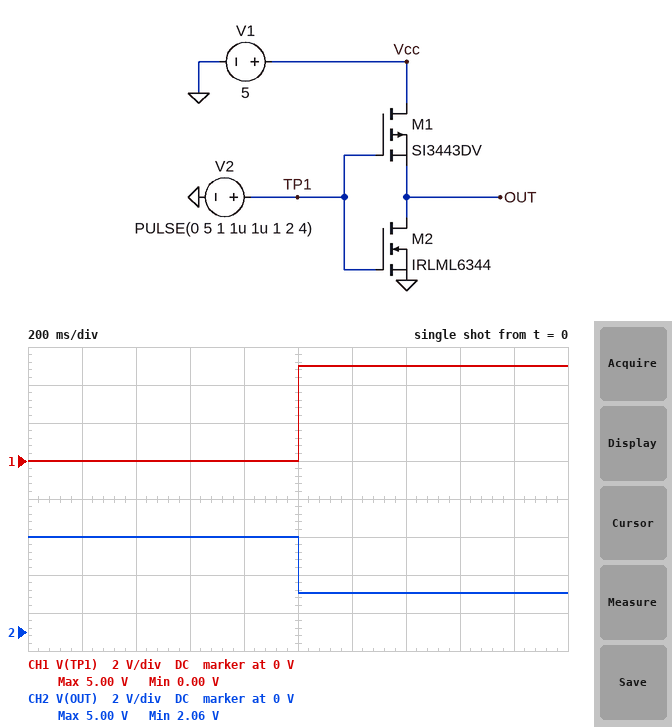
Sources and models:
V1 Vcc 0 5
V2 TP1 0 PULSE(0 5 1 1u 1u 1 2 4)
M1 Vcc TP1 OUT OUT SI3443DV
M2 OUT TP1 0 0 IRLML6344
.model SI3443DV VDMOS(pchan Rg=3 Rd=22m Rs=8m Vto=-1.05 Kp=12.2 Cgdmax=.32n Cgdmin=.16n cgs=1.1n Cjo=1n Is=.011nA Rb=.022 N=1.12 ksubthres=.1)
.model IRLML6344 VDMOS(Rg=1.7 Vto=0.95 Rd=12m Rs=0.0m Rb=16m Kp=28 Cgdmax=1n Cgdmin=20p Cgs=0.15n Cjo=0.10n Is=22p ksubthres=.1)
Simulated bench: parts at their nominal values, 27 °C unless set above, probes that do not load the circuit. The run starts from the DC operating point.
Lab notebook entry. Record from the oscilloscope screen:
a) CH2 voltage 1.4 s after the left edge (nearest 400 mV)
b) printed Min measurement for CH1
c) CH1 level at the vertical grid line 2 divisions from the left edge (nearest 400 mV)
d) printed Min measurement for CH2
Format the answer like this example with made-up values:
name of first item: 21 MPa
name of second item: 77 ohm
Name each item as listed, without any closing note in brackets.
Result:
CH2 voltage 1.4 s after the left edge: 2.0 V
printed Min measurement for CH1: 0.00 V
CH1 level at the vertical grid line 2 divisions from the left edge: 0 V
printed Min measurement for CH2: 2.06 V
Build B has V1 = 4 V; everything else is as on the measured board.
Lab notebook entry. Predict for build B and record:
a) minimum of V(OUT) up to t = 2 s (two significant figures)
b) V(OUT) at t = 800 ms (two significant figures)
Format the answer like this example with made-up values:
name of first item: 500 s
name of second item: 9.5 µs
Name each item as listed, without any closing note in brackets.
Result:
minimum of V(OUT) up to t = 2 s: 1.6 V
V(OUT) at t = 800 ms: 4.0 V
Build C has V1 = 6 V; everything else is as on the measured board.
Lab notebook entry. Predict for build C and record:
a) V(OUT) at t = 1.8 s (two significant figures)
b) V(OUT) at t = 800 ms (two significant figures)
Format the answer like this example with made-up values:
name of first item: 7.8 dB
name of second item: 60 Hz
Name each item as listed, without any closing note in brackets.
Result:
V(OUT) at t = 1.8 s: 2.6 V
V(OUT) at t = 800 ms: 6.0 V
